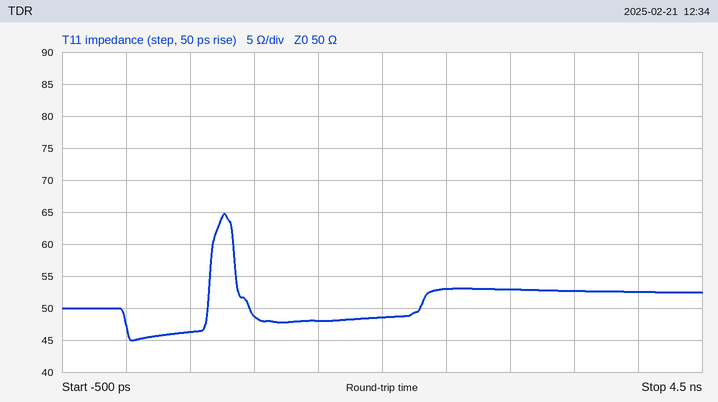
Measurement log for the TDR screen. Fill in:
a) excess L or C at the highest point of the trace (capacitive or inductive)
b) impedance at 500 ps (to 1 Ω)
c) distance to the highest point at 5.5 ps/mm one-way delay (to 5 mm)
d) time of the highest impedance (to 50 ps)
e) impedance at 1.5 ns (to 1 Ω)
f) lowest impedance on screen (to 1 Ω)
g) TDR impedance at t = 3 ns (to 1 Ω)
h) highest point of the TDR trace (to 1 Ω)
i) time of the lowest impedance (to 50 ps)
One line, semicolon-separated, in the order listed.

inductive; 46 Ω; 70 mm; 750 ps; 48 Ω; 45 Ω; 53 Ω; 65 Ω; 50 ps
